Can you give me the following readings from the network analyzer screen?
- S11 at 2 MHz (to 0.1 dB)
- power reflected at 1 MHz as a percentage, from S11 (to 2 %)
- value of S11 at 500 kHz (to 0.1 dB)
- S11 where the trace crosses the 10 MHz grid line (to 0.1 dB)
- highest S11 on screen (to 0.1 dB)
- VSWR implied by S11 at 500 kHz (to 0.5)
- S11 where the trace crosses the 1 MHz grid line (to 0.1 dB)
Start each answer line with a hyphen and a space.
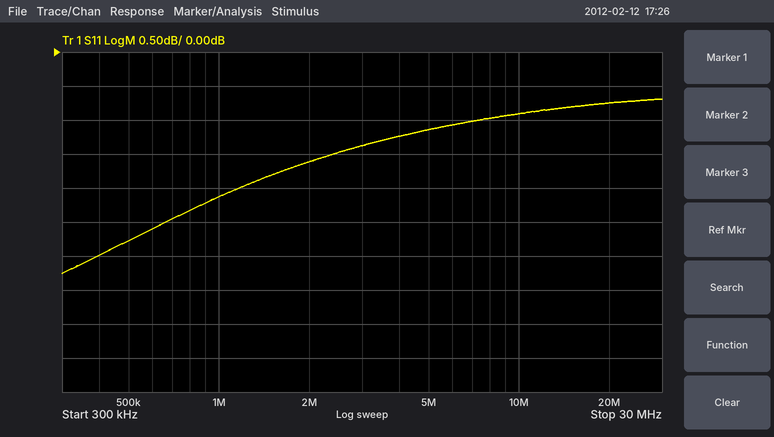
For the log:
- -1.6 dB
- 62 %
- -2.8 dB
- -0.9 dB
- -0.7 dB
- 6.5
- -2.1 dB
